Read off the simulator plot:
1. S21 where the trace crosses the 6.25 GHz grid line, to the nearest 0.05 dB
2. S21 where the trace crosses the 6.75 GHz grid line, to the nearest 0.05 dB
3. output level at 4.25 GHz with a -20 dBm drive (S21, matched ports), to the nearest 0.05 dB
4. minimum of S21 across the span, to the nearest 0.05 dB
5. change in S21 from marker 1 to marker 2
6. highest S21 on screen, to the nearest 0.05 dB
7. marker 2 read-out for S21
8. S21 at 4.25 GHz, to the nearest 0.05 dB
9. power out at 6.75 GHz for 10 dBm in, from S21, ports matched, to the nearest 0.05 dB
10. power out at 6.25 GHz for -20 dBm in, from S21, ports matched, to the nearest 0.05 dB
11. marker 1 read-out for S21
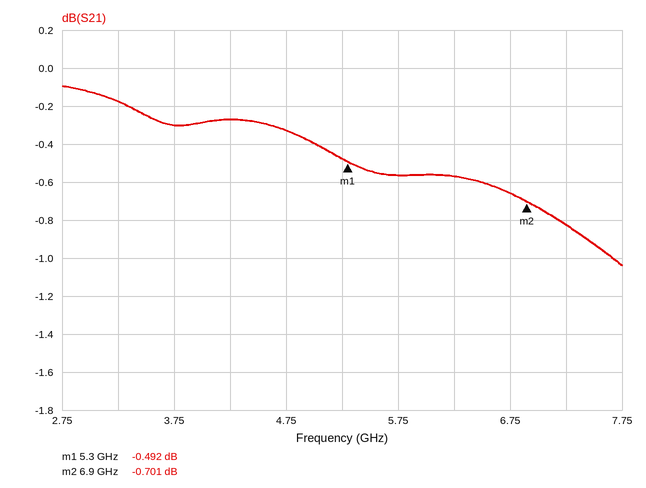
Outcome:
-0.55 dB
-0.65 dB
-20.25 dBm
-1.05 dB
-0.209 dB
-0.10 dB
-0.701 dB
-0.25 dB
9.35 dBm
-20.55 dBm
-0.492 dB
